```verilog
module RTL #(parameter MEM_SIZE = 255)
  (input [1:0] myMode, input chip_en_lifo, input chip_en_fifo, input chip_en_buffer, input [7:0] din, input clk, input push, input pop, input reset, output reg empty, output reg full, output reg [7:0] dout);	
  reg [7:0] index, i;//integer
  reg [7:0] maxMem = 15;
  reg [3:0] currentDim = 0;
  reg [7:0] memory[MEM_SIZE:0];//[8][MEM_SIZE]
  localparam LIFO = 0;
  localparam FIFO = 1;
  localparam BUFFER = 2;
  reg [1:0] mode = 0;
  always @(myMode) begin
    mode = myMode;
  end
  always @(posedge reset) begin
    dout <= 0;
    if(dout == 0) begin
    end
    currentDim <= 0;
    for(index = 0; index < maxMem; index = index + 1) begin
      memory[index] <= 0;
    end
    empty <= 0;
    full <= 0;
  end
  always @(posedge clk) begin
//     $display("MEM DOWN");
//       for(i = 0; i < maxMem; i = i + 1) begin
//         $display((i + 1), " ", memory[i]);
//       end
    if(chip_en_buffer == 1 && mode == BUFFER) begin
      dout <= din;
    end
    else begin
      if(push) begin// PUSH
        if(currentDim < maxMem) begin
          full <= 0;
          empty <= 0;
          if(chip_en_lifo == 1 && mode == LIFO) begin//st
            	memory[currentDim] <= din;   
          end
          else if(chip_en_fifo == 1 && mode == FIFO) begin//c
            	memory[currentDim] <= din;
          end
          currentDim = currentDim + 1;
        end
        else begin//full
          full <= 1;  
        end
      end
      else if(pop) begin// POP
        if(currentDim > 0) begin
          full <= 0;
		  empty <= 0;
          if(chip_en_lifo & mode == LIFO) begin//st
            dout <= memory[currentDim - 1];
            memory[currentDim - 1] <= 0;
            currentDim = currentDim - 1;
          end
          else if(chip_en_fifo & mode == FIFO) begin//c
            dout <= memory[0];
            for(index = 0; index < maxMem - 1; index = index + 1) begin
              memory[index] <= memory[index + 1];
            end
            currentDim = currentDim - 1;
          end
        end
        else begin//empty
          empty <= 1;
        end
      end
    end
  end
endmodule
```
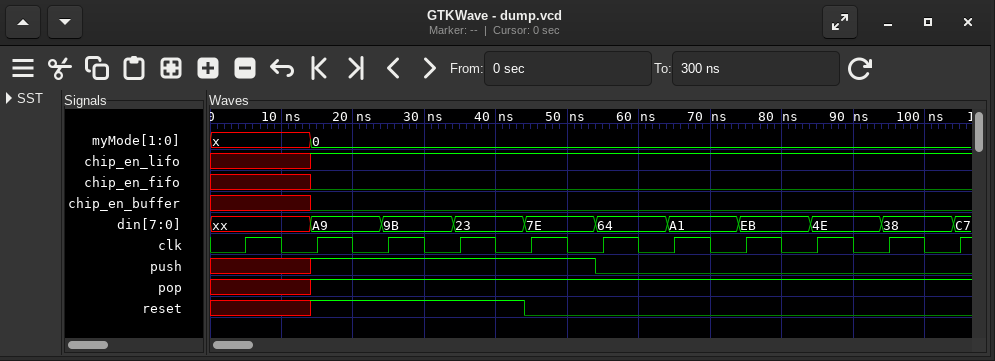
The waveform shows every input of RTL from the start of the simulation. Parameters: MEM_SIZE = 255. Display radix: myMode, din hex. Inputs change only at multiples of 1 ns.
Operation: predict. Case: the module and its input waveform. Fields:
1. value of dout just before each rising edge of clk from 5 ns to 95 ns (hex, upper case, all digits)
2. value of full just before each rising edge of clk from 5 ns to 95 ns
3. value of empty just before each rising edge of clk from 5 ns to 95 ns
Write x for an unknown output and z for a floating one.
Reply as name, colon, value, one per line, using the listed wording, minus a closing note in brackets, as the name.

value of dout just before each rising edge of clk from 5 ns to 95 ns: x, 00, 00, 00, 00, 00, 7E, 23, 9B, A9
value of full just before each rising edge of clk from 5 ns to 95 ns: x 0 0 0 0 0 0 0 0 0
value of empty just before each rising edge of clk from 5 ns to 95 ns: x 0 0 0 0 0 0 0 0 0
